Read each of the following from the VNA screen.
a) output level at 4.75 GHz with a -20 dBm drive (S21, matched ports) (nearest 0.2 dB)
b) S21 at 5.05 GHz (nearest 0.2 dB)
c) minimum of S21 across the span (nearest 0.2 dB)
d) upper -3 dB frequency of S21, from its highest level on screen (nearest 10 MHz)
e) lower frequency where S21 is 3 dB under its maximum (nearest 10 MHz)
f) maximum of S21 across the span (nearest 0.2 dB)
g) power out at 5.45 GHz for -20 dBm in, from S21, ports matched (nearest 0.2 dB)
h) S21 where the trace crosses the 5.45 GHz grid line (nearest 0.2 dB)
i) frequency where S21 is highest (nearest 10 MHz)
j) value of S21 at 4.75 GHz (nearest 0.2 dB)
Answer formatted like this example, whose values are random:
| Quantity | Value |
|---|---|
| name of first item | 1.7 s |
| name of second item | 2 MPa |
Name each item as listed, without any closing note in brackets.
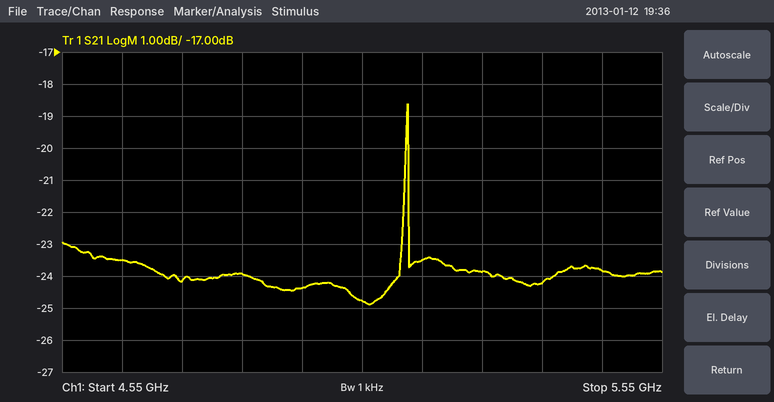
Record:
| Quantity | Value |
|---|---|
| output level at 4.75 GHz with a -20 dBm drive (S21, matched ports) | -44.2 dBm |
| S21 at 5.05 GHz | -24.8 dB |
| minimum of S21 across the span | -24.8 dB |
| upper -3 dB frequency of S21, from its highest level on screen | 5.13 GHz |
| lower frequency where S21 is 3 dB under its maximum | 5.12 GHz |
| maximum of S21 across the span | -18.6 dB |
| power out at 5.45 GHz for -20 dBm in, from S21, ports matched | -43.8 dBm |
| S21 where the trace crosses the 5.45 GHz grid line | -23.8 dB |
| frequency where S21 is highest | 5.13 GHz |
| value of S21 at 4.75 GHz | -24.2 dB |
